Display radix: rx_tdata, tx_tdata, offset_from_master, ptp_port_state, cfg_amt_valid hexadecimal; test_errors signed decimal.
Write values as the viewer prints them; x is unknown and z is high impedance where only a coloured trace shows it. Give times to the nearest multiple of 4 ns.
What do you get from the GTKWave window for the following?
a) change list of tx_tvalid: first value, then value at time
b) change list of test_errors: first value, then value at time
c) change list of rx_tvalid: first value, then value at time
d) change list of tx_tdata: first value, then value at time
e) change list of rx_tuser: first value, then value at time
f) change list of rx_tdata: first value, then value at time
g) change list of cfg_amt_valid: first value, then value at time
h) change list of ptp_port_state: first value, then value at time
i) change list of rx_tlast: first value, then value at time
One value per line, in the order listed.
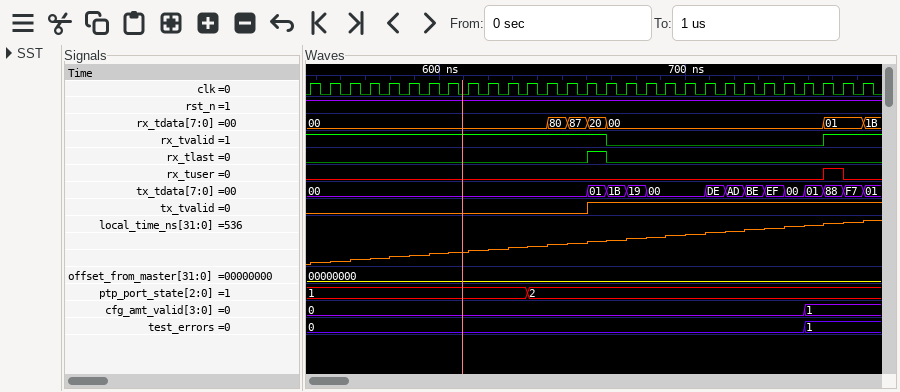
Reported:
0, 1 at 660 ns
0, 1 at 748 ns
1, 0 at 668 ns, 1 at 756 ns
00, 01 at 660 ns, 1B at 668 ns, 19 at 676 ns, 00 at 684 ns, DE at 708 ns, AD at 716 ns, BE at 724 ns, EF at 732 ns, 00 at 740 ns, 01 at 748 ns, 88 at 756 ns, F7 at 764 ns, 01 at 772 ns
0, 1 at 756 ns, 0 at 764 ns
00, 80 at 644 ns, 87 at 652 ns, 20 at 660 ns, 00 at 668 ns, 01 at 756 ns, 1B at 772 ns
0, 1 at 748 ns
1, 2 at 636 ns
0, 1 at 660 ns, 0 at 668 ns
